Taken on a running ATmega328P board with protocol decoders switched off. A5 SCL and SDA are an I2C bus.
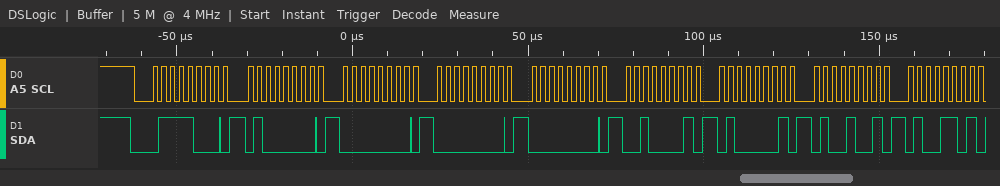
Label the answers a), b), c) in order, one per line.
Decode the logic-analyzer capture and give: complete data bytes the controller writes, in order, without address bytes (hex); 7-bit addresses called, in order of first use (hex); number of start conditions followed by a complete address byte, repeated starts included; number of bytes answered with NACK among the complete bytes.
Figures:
a) 40 00 00 00 21 41 49 4D
b) 0x3C
c) 1
d) 0
